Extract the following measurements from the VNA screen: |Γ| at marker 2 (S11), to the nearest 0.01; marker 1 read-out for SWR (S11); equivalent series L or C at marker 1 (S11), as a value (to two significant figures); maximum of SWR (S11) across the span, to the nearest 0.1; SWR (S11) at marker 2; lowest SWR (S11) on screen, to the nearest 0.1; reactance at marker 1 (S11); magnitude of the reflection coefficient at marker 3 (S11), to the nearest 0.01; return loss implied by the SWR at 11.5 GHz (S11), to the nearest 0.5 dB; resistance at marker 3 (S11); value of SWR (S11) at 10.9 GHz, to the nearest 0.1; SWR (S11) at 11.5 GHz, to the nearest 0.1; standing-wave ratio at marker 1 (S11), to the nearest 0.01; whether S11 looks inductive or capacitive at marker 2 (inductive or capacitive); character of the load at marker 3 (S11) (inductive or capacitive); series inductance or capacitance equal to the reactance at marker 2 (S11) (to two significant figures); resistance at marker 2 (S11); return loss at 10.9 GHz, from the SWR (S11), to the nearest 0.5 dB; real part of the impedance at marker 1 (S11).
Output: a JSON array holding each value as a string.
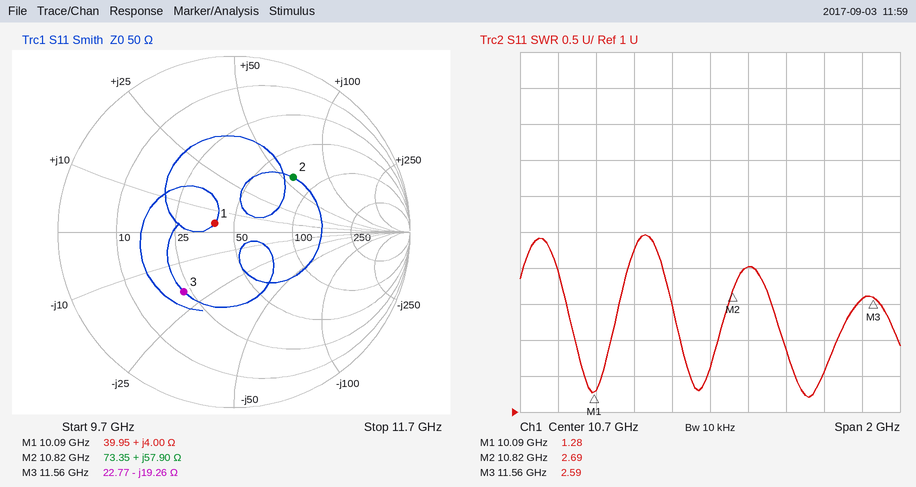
["0.46", "1.28", "63 pH", "3.5", "2.69", "1.2", "+4.00 Ω", "0.44", "7.0 dB", "22.77 Ω", "3.0", "2.6", "1.27", "inductive", "capacitive", "850 pH", "73.35 Ω", "6.0 dB", "39.95 Ω"]
